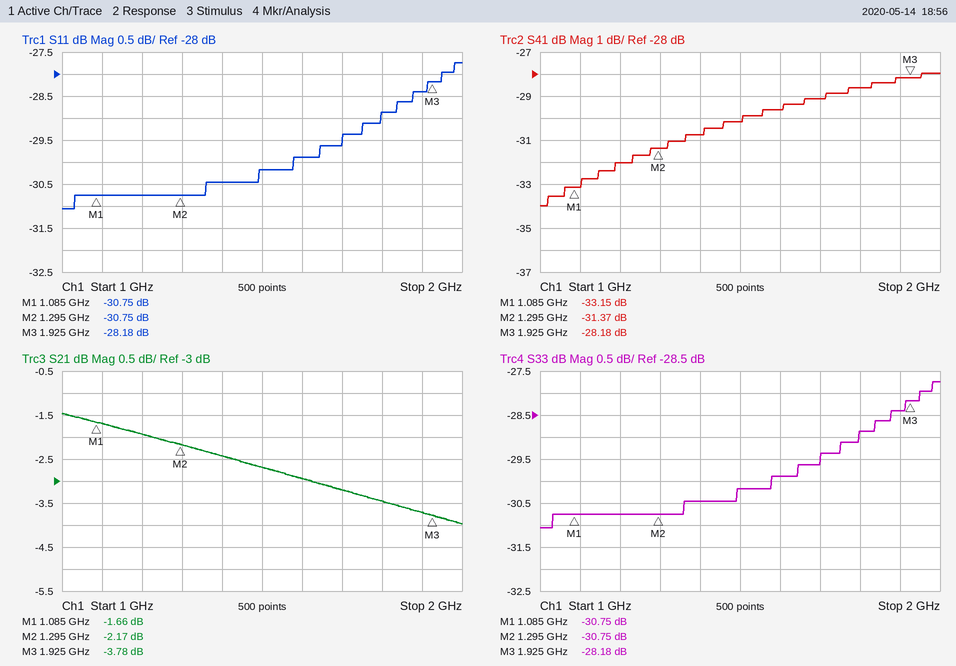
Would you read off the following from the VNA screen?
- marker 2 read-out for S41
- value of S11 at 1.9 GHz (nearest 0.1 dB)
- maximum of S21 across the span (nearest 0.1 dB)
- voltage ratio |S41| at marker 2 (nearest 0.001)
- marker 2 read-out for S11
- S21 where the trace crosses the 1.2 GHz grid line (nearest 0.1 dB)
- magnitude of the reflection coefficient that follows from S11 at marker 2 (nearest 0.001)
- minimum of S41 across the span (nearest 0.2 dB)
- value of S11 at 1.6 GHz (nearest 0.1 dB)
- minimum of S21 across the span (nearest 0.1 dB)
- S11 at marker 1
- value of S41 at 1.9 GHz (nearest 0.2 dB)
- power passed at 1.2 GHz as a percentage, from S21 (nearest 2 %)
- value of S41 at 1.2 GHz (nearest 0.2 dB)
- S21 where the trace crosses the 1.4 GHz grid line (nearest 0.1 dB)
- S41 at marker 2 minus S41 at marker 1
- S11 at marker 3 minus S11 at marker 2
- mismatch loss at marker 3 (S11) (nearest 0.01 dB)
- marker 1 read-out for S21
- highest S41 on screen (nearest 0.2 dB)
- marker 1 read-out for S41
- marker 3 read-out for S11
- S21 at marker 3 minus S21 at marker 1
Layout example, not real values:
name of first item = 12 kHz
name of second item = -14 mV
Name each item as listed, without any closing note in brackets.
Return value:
marker 2 read-out for S41 = -31.37 dB
value of S11 at 1.9 GHz = -28.4 dB
maximum of S21 across the span = -1.5 dB
voltage ratio |S41| at marker 2 = 0.027
marker 2 read-out for S11 = -30.75 dB
S21 where the trace crosses the 1.2 GHz grid line = -1.9 dB
magnitude of the reflection coefficient that follows from S11 at marker 2 = 0.029
minimum of S41 across the span = -34.0 dB
value of S11 at 1.6 GHz = -29.9 dB
minimum of S21 across the span = -4.0 dB
S11 at marker 1 = -30.75 dB
value of S41 at 1.9 GHz = -28.2 dB
power passed at 1.2 GHz as a percentage, from S21 = 64 %
value of S41 at 1.2 GHz = -32.0 dB
S21 where the trace crosses the 1.4 GHz grid line = -2.4 dB
S41 at marker 2 minus S41 at marker 1 = 1.78 dB
S11 at marker 3 minus S11 at marker 2 = 2.57 dB
mismatch loss at marker 3 (S11) = 0.01 dB
marker 1 read-out for S21 = -1.66 dB
highest S41 on screen = -28.0 dB
marker 1 read-out for S41 = -33.15 dB
marker 3 read-out for S11 = -28.18 dB
S21 at marker 3 minus S21 at marker 1 = -2.12 dB
